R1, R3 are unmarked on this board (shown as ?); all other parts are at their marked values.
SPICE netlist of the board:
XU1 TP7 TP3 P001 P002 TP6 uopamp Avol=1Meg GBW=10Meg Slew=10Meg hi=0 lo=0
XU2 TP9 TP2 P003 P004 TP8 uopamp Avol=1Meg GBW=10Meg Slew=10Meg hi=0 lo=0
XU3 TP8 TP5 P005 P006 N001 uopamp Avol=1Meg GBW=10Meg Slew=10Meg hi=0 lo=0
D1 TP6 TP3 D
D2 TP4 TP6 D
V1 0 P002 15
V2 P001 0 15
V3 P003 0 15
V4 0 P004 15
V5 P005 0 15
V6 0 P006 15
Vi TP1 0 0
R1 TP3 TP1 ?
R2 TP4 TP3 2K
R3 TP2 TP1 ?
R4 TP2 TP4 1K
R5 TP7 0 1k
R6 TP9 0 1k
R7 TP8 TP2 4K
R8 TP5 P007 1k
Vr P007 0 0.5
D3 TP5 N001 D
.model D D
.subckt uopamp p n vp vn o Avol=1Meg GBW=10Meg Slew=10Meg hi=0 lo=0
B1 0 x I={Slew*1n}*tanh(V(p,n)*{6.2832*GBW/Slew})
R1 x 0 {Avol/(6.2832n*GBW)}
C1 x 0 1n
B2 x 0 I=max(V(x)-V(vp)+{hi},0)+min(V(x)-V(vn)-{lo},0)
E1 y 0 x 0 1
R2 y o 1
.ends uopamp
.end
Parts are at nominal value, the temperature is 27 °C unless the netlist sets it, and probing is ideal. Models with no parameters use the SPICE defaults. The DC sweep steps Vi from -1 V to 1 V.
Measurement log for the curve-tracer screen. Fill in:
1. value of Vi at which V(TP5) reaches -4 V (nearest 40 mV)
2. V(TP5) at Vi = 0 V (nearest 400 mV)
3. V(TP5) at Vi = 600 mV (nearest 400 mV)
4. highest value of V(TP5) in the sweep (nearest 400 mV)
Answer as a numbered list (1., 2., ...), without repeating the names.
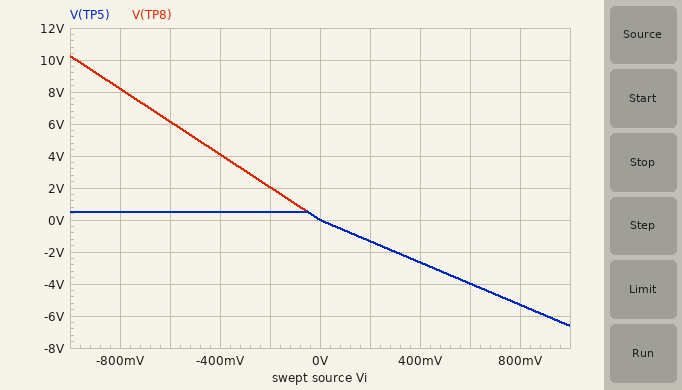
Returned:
1. 600 mV
2. 0 V
3. -4.0 V
4. 400 mV
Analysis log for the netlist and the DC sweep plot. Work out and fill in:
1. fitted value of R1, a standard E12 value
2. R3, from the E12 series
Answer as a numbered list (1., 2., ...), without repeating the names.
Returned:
1. 2.2 kΩ
2. 390 Ω
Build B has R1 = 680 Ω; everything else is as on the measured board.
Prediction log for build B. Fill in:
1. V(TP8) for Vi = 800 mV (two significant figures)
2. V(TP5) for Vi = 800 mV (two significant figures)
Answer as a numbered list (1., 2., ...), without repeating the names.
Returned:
1. 1.2 V
2. 500 mV
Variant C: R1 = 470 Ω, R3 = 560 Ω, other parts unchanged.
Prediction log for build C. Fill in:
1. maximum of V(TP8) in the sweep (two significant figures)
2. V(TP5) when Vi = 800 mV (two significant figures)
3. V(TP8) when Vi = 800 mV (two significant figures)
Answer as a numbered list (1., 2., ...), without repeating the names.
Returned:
1. 9.9 V
2. 500 mV
3. 7.9 V
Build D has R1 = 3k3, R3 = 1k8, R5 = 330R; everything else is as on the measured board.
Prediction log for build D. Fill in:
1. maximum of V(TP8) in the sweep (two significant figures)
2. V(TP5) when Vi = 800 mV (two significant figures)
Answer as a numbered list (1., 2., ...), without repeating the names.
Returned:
1. 2.2 V
2. 160 mV
